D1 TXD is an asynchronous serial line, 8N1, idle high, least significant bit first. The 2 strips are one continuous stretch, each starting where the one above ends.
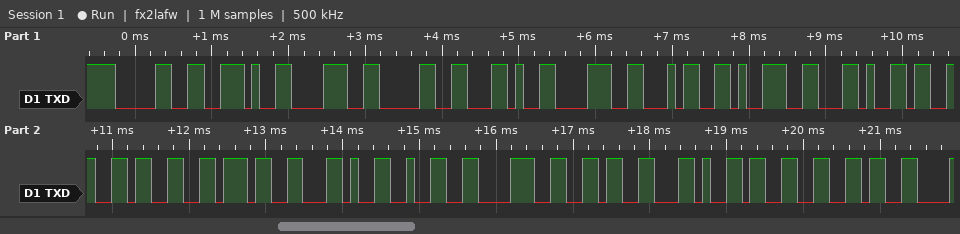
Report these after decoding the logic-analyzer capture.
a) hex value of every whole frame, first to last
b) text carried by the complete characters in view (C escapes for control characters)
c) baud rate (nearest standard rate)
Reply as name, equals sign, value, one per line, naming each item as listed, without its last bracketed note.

hex value of every whole frame, first to last = 30 2E 38 30 2C 38 34 39 2C 33 33 37 2C 32 38 36 2C 33 36
text carried by the complete characters in view = "0.80,849,337,286,36"
baud rate = 9600 baud
